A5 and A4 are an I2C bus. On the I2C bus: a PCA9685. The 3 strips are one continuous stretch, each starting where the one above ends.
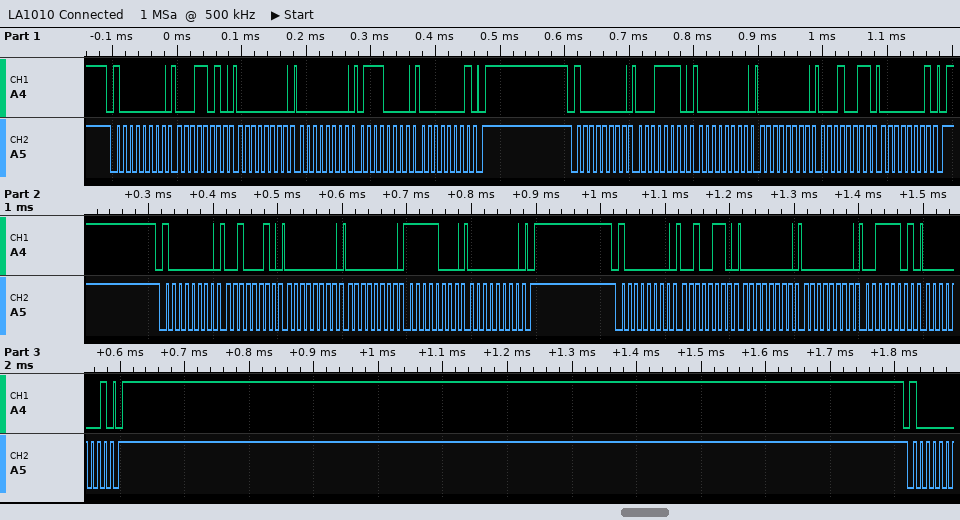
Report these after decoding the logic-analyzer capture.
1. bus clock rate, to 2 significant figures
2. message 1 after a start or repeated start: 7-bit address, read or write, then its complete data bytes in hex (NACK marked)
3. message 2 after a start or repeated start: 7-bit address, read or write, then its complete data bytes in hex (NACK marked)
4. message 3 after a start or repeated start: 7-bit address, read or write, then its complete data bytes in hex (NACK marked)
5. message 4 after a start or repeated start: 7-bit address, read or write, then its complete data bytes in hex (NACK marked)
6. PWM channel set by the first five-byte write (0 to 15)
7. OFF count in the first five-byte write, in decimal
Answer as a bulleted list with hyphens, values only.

- 100 kHz
- 0x40 write: 1A 00 00 70 01
- 0x40 write: 1E 00 00 13 01
- 0x40 write: 22 00 00 F8 00
- 0x40 write: 26 00 00 3D 01
- 5
- 368
